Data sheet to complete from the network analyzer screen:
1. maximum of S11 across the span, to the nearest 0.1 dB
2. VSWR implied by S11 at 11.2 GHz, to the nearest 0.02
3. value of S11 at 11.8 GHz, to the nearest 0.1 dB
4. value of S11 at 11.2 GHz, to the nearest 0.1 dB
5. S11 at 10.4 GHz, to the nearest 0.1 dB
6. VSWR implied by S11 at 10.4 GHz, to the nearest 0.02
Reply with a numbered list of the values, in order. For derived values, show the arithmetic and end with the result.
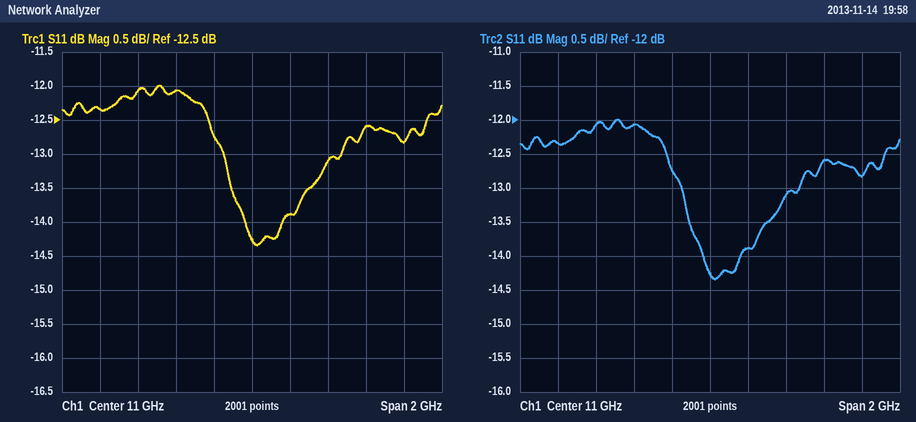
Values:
1. -12.0 dB
2. |Γ| = 10^(-13.9/20) = 0.2018; VSWR = (1 + 0.2018)/(1 − 0.2018) ≈ 1.51, so 1.50 to the nearest 0.02
3. -12.8 dB
4. -13.9 dB
5. -12.1 dB
6. |Γ| = 10^(-12.1/20) = 0.2483; VSWR = (1 + 0.2483)/(1 − 0.2483) ≈ 1.66
